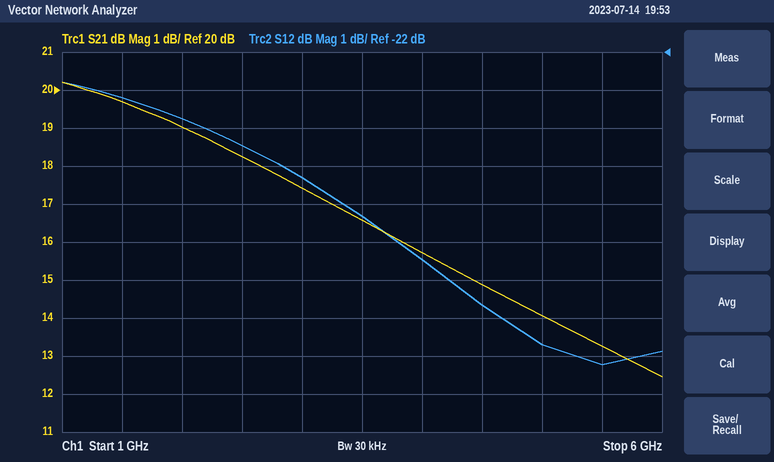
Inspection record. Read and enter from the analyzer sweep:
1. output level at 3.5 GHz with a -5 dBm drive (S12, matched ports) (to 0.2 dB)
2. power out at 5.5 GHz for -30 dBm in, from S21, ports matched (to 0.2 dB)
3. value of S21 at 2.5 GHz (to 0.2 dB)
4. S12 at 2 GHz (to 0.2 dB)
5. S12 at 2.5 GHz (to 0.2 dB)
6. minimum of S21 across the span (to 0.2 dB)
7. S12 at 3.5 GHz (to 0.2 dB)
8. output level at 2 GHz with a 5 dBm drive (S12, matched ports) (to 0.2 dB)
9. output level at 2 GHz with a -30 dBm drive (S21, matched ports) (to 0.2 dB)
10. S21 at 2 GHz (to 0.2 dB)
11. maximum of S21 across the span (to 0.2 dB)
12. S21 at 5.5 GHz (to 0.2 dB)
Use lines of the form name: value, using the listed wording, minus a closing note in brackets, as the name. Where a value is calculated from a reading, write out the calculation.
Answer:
output level at 3.5 GHz with a -5 dBm drive (S12, matched ports): -5 dBm + (-26.4 dB) = -31.4 dBm
power out at 5.5 GHz for -30 dBm in, from S21, ports matched: -30 dBm + (13.2 dB) = -16.8 dBm
value of S21 at 2.5 GHz: 18.2 dB
S12 at 2 GHz: -23.8 dB
S12 at 2.5 GHz: -24.4 dB
minimum of S21 across the span: 12.4 dB
S12 at 3.5 GHz: -26.4 dB
output level at 2 GHz with a 5 dBm drive (S12, matched ports): 5 dBm + (-23.8 dB) = -18.8 dBm
output level at 2 GHz with a -30 dBm drive (S21, matched ports): -30 dBm + (19.0 dB) = -11.0 dBm
S21 at 2 GHz: 19.0 dB
maximum of S21 across the span: 20.2 dB
S21 at 5.5 GHz: 13.2 dB
